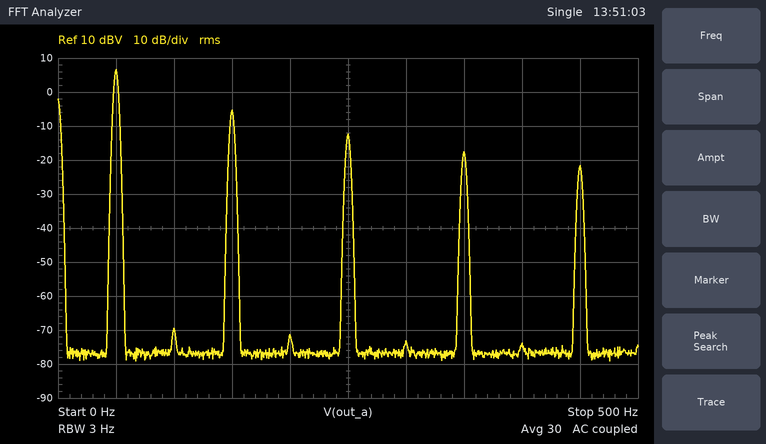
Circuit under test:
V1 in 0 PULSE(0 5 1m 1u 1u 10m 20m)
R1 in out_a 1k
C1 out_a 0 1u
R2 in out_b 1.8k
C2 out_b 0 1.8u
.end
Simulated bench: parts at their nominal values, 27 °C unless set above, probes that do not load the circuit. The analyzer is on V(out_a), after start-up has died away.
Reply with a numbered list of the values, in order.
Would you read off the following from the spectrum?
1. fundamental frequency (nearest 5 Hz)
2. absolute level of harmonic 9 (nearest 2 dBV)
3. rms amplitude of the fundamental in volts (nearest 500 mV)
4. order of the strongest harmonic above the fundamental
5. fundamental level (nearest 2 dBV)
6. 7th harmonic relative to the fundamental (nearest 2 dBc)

1. 50 Hz
2. -22 dBV
3. 2.0 V
4. 3
5. 6 dBV
6. -24 dBc
